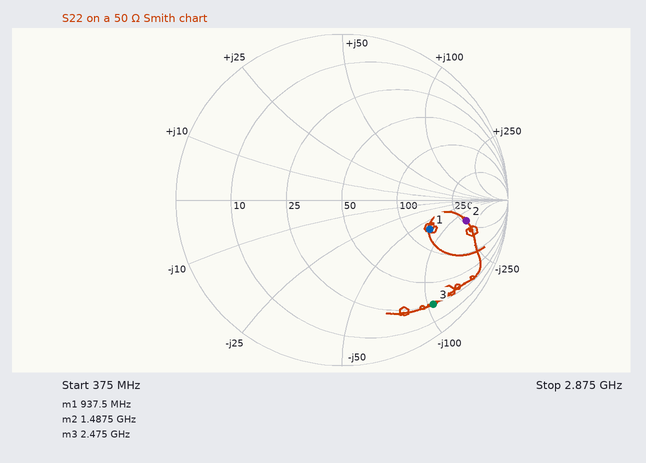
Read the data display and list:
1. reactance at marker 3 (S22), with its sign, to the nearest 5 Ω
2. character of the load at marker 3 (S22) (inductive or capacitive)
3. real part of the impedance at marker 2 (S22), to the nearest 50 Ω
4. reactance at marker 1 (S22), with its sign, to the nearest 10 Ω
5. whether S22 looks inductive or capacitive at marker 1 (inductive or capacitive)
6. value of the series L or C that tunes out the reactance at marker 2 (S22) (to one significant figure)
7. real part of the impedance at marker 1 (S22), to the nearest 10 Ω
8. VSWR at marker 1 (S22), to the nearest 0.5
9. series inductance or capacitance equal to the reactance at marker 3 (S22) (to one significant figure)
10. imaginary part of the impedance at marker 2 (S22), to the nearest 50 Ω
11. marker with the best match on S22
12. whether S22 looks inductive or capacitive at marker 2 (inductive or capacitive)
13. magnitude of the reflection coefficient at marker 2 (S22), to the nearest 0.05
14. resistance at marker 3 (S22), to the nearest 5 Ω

-105 Ω
capacitive
250 Ω
-70 Ω
capacitive
20 nH
140 Ω
3.5
600 fF
-150 Ω
marker 1
capacitive
0.75
25 Ω
